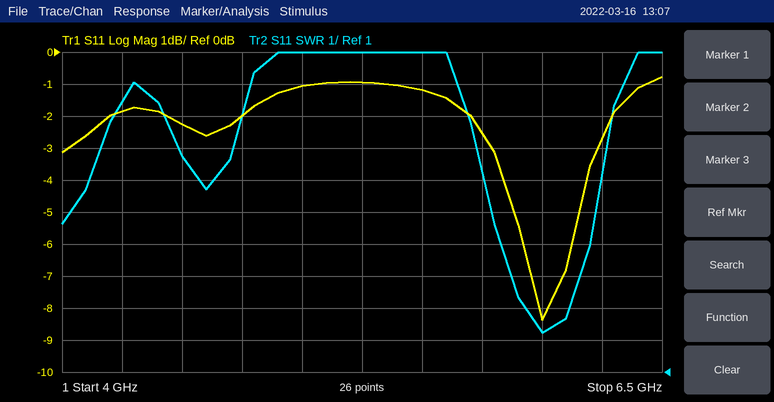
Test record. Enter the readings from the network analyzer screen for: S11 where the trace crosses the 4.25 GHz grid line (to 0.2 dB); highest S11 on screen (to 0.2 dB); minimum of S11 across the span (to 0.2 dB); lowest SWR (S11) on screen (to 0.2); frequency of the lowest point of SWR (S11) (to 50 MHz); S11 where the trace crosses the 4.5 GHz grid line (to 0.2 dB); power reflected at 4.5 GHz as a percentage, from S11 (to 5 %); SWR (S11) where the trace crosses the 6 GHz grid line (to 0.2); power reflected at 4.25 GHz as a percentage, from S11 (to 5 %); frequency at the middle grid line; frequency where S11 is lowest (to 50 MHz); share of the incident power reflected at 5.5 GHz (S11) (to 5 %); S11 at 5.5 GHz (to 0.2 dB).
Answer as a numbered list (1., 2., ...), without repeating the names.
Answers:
1. -1.8 dB
2. -0.8 dB
3. -8.4 dB
4. 2.2
5. 6.00 GHz
6. -2.2 dB
7. 60 %
8. 2.2
9. 65 %
10. 5.25 GHz
11. 6.00 GHz
12. 75 %
13. -1.2 dB
